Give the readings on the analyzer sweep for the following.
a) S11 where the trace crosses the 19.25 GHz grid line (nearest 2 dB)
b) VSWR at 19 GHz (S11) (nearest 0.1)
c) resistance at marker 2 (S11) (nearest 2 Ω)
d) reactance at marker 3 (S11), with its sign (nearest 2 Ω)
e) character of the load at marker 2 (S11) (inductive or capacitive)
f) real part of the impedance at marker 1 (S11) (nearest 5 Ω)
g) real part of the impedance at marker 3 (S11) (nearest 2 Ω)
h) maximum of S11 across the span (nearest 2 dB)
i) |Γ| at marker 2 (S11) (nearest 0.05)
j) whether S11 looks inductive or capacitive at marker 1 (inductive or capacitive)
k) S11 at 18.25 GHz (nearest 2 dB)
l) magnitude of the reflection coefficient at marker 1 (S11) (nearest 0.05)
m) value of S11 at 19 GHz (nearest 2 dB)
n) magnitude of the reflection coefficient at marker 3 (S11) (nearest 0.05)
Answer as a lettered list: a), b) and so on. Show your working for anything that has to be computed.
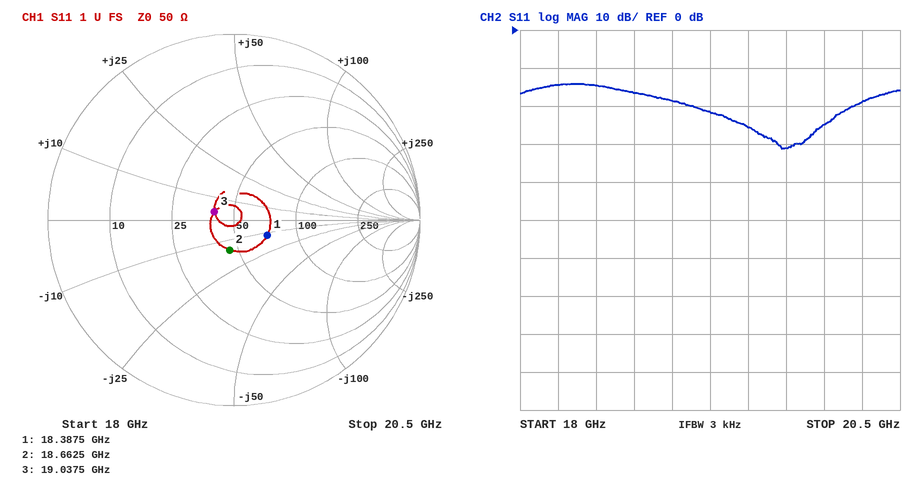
a) -22 dB
b) |Γ| = 10^(-18/20) = 0.1259; VSWR = (1 + 0.1259)/(1 − 0.1259) ≈ 1.3
c) 46 Ω
d) +4 Ω
e) capacitive
f) 70 Ω
g) 40 Ω
h) -14 dB
i) 0.15
j) capacitive
k) -14 dB
l) 0.20
m) -18 dB
n) 0.10
